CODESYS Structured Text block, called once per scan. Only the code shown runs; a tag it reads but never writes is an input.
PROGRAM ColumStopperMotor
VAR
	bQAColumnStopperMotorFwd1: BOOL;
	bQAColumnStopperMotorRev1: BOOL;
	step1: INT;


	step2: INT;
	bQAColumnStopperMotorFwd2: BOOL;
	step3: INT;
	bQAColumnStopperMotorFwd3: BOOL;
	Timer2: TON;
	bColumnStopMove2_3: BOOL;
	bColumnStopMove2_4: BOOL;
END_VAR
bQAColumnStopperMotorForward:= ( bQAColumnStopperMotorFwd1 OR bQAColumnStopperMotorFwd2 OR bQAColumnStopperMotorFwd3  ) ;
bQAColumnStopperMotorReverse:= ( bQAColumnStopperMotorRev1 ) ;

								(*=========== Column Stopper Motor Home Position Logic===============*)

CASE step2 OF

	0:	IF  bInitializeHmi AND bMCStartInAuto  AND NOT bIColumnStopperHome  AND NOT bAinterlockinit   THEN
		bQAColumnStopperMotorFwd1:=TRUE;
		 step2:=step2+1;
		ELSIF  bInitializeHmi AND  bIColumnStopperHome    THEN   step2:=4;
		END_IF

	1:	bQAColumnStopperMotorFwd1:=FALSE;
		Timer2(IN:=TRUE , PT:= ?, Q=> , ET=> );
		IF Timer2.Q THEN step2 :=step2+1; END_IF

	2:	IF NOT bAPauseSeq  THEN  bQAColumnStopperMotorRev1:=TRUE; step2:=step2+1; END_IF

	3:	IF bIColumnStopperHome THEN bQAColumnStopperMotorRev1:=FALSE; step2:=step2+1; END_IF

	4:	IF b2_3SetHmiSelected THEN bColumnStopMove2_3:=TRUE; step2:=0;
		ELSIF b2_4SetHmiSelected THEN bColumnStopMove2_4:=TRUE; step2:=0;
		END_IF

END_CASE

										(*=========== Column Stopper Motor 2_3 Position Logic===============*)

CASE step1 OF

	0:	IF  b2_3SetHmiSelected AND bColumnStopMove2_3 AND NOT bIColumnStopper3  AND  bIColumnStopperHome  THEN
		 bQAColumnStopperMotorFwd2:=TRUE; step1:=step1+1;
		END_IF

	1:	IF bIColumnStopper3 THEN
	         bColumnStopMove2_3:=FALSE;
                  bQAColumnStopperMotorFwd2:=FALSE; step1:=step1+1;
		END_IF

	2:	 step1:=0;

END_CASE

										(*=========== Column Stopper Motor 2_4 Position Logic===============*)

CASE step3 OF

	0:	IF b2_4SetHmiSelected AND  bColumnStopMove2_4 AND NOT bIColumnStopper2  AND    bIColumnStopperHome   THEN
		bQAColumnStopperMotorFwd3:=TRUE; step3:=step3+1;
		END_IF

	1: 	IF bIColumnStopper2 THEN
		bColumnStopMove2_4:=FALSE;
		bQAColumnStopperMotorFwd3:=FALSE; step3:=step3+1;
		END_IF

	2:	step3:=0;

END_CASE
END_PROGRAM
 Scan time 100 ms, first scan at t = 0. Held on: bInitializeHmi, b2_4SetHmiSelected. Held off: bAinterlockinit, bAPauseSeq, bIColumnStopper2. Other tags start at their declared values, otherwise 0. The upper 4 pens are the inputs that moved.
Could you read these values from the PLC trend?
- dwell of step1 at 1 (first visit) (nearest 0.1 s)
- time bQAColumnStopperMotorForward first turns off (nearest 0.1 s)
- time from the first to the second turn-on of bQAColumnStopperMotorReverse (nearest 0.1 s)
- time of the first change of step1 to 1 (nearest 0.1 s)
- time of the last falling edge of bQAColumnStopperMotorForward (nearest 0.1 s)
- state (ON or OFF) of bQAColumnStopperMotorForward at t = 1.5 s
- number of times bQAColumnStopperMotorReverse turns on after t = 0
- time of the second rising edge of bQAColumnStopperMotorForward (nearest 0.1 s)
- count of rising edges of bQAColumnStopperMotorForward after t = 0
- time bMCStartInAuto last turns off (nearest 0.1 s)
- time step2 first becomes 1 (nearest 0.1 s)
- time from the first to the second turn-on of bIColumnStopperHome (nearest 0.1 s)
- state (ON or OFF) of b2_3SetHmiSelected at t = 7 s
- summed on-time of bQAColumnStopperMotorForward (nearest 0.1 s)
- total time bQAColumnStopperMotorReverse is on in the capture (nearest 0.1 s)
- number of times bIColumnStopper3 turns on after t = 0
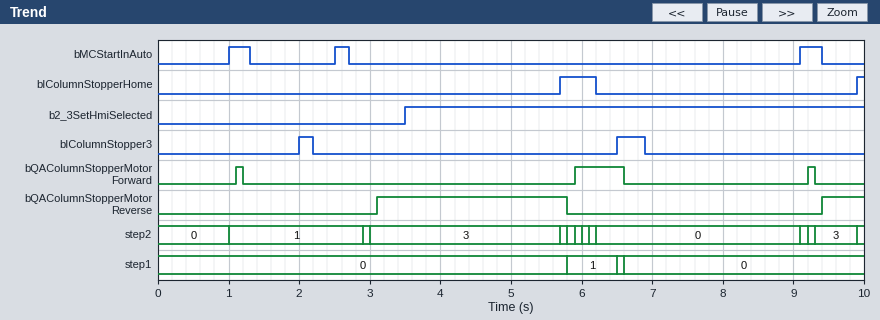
0.7 s
1.2 s
6.3 s
5.8 s
9.3 s
OFF
2
5.9 s
3
9.4 s
1.0 s
4.2 s
ON
0.9 s
3.3 s
2
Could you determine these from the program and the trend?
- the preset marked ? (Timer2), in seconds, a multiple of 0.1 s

1.8 s
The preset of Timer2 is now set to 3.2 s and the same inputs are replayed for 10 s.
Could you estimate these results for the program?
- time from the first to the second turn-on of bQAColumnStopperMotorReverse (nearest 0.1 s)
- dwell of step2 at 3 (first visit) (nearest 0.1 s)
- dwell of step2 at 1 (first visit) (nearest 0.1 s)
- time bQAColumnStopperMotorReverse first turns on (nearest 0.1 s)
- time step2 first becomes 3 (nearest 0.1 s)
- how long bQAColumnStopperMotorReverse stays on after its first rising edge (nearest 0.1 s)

4.9 s
1.3 s
3.3 s
4.5 s
4.4 s
1.3 s
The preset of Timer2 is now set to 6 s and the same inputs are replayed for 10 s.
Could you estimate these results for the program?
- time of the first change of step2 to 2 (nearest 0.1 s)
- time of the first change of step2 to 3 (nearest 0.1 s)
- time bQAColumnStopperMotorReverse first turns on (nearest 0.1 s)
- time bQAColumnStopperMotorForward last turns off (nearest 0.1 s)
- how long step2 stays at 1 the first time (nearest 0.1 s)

7.1 s
7.2 s
7.3 s
1.2 s
6.1 s
